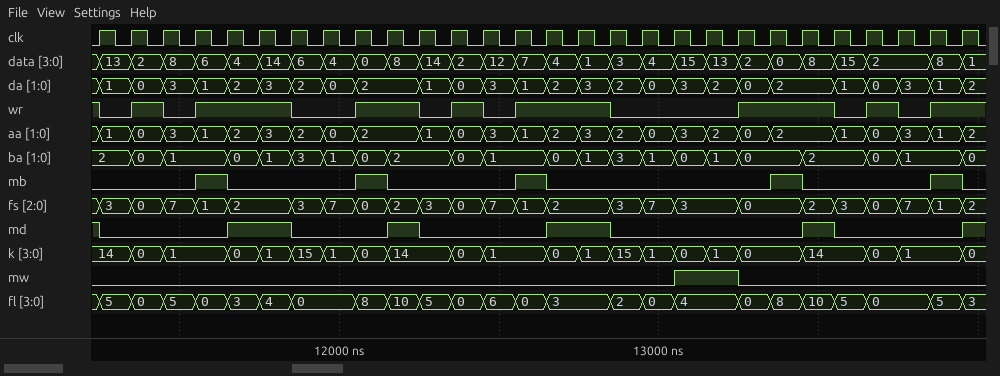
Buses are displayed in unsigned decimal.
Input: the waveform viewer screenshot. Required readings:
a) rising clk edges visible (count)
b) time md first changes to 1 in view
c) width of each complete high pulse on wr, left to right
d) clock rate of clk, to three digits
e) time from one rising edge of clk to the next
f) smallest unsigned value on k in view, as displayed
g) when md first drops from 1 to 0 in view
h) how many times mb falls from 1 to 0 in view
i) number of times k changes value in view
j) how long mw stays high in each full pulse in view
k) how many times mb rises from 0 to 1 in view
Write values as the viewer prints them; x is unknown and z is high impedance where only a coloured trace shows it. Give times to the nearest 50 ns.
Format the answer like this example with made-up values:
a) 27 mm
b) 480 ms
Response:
a) 28
b) 11650 ns
c) 100 ns, 300 ns, 200 ns, 100 ns, 300 ns, 300 ns, 100 ns
d) 10.0 MHz
e) 100 ns
f) 0
g) 11250 ns
h) 5
i) 21
j) 200 ns
k) 5
